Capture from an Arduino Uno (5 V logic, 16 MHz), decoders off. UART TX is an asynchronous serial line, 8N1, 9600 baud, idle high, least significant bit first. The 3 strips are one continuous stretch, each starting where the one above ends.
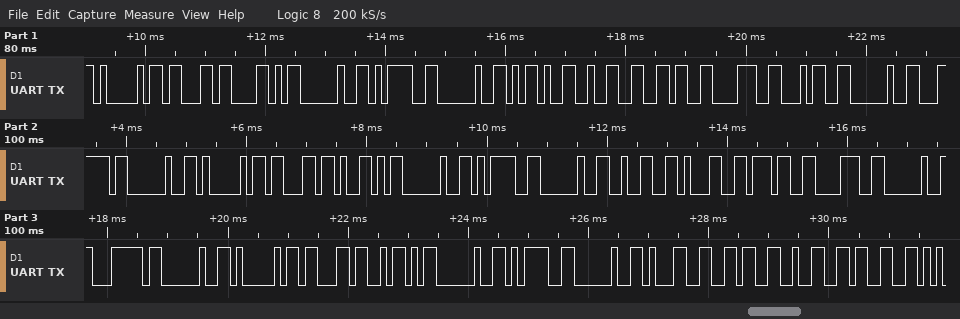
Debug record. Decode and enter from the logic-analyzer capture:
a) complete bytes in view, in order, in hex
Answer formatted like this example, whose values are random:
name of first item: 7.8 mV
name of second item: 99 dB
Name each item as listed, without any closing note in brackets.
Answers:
complete bytes in view, in order, in hex: 41 63 58 20 3D 20 2D 32 36 38 34 20 7C 20 41 63 59 20 3D 20 32 31 37 38 20 7C 20 41 63 5A 20 3D 20 31 36 32 33
